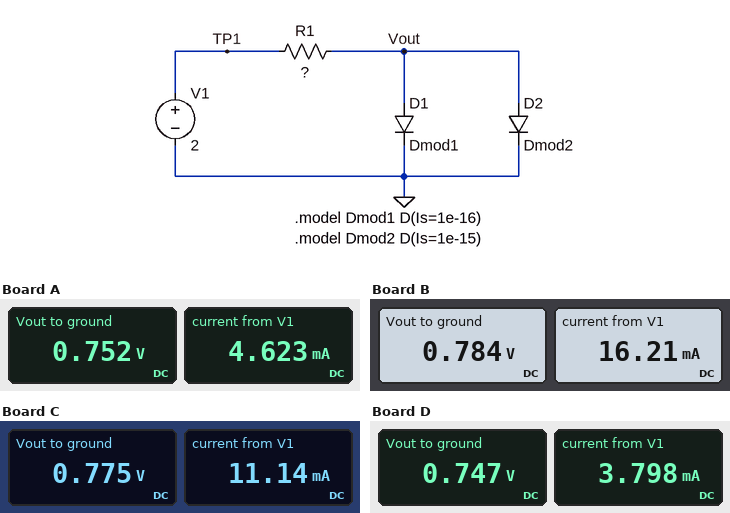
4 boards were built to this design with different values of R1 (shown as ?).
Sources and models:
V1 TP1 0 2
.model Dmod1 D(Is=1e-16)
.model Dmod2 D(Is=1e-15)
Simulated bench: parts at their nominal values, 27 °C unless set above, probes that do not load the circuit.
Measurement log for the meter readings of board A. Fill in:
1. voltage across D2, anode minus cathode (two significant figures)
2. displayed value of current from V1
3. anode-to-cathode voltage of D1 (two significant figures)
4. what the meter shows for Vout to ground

750 mV
4.623 mA
750 mV
0.752 V
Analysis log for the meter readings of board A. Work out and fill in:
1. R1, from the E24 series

270 Ω
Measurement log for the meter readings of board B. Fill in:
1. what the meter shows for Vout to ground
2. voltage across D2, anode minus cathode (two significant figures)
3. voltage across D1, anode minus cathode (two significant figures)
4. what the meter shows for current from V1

0.784 V
780 mV
780 mV
16.21 mA
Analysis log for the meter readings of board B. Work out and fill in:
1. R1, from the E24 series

75 Ω
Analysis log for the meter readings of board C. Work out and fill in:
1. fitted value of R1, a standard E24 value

110 Ω
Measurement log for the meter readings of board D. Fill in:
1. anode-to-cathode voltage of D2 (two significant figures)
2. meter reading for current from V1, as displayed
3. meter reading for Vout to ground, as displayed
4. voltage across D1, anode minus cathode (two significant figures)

750 mV
3.798 mA
0.747 V
750 mV
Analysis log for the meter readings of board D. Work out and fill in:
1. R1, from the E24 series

330 Ω
